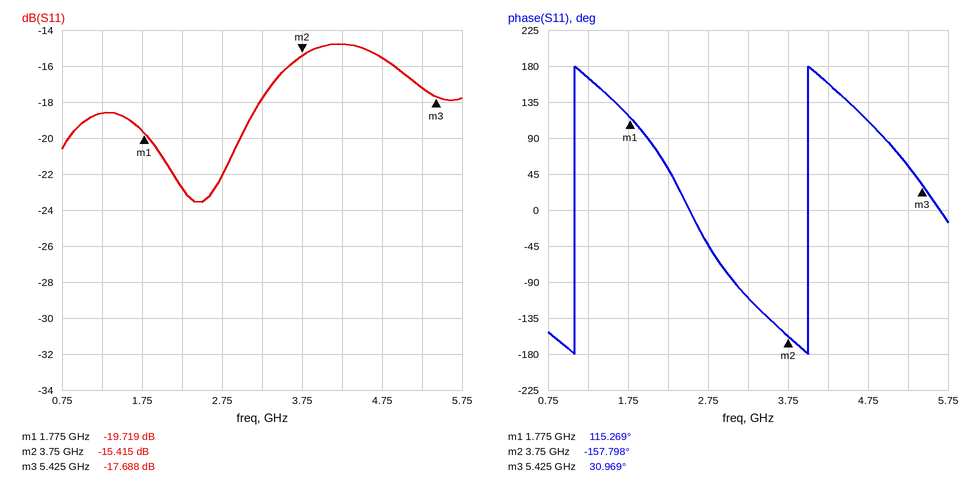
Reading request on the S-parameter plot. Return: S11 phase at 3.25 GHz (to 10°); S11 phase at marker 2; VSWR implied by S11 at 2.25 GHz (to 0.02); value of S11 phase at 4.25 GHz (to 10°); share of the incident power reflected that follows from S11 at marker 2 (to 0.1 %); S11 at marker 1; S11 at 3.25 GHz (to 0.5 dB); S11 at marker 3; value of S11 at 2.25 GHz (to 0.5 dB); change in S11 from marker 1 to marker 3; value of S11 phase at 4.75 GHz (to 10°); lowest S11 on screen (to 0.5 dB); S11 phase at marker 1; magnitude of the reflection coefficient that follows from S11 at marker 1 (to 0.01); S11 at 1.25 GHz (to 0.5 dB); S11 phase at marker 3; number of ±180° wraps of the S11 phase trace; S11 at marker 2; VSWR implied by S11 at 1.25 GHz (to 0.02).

-110°
-157.798°
1.16
160°
2.9 %
-19.719 dB
-18.0 dB
-17.688 dB
-23.0 dB
2.031 dB
110°
-23.5 dB
115.269°
0.10
-18.5 dB
30.969°
2
-15.415 dB
1.26
